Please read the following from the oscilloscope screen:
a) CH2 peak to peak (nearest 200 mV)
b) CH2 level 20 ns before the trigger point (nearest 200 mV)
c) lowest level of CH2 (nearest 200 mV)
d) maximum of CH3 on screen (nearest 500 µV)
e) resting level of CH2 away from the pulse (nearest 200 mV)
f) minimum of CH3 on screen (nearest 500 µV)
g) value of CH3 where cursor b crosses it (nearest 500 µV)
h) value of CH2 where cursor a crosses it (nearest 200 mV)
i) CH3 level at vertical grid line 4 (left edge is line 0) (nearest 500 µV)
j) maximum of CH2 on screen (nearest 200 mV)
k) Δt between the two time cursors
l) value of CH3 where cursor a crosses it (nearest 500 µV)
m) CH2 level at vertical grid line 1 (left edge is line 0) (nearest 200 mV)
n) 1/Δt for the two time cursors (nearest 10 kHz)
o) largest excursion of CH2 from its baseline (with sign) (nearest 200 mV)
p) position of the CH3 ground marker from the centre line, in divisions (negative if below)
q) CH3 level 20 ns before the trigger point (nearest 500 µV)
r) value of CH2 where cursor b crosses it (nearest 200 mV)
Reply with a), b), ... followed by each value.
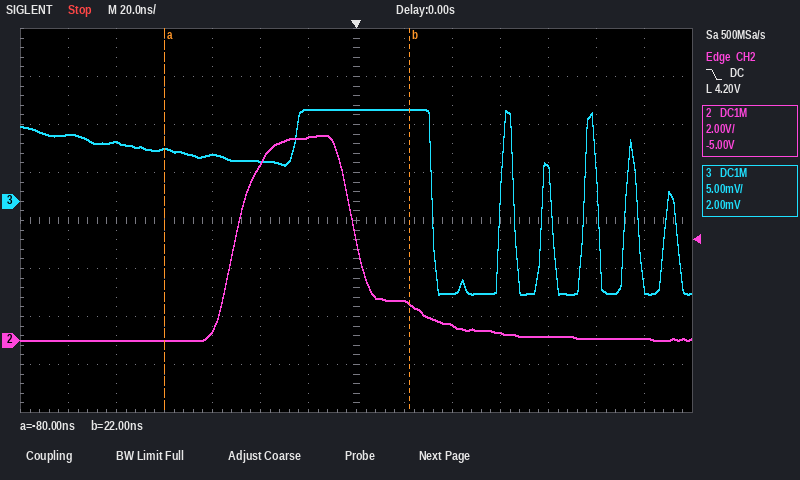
a) 8.6 V
b) 8.4 V
c) 0.0 V
d) 9.5 mV
e) 0.0 V
f) -9.5 mV
g) 9.5 mV
h) 0.0 V
i) 5.0 mV
j) 8.6 V
k) 102 ns
l) 5.5 mV
m) 0.0 V
n) 9.80 MHz
o) +8.6 V
p) +0.4 div
q) 9.5 mV
r) 1.6 V
